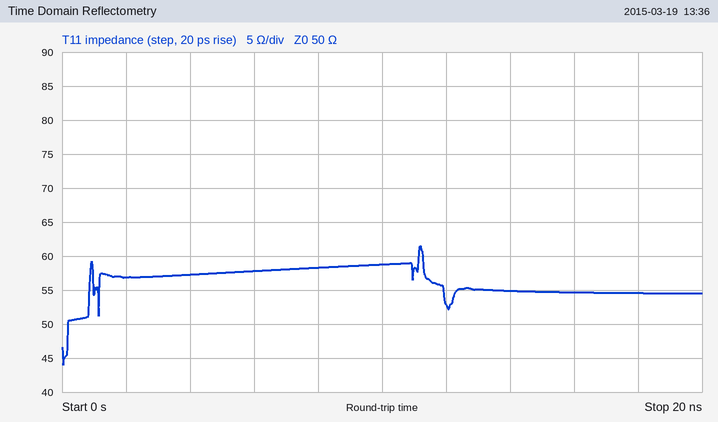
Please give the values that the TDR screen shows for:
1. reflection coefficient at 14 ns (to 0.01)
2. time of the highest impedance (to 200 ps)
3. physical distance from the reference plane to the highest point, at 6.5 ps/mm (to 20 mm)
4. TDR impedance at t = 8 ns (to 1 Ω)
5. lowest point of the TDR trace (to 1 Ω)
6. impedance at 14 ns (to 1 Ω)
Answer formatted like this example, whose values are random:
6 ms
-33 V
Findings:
+0.05
11.2 ns
860 mm
58 Ω
44 Ω
55 Ω
